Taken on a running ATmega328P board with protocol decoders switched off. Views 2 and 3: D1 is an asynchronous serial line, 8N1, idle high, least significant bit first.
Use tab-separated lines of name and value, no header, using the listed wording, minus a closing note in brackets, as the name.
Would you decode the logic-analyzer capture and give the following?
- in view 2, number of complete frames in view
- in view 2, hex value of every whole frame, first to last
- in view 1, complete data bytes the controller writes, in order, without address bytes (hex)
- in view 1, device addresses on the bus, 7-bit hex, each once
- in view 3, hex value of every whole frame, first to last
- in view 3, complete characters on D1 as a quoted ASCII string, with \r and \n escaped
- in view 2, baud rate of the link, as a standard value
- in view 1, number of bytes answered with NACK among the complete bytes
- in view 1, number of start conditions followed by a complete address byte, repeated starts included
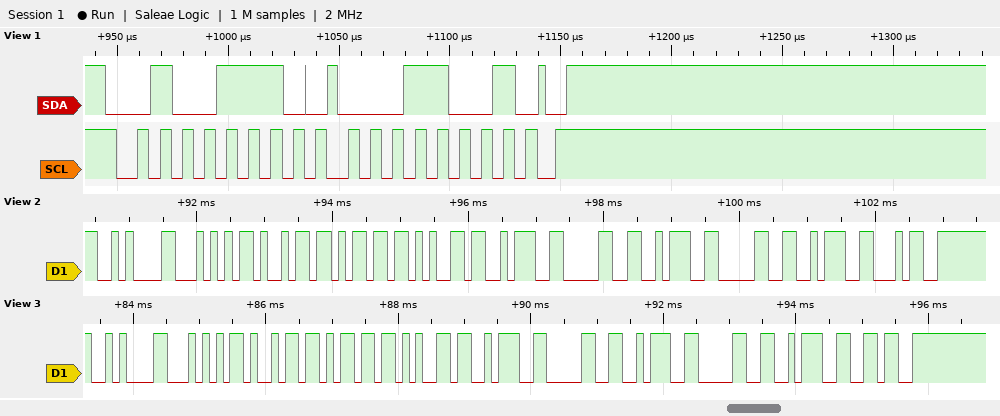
in view 2, number of complete frames in view	11
in view 2, hex value of every whole frame, first to last	0x0A 0x54 0x69 0x6D 0x65 0x3A 0x30 0x3A 0x30 0x3A 0x34
in view 1, complete data bytes the controller writes, in order, without address bytes	19
in view 1, device addresses on the bus, 7-bit hex, each once	0x27
in view 3, hex value of every whole frame, first to last	0x0A 0x54 0x69 0x6D 0x65 0x3A 0x30 0x3A 0x30 0x3A 0x36
in view 3, complete characters on D1 as a quoted ASCII string, with \r and \n escaped	"\nTime:0:0:6"
in view 2, baud rate of the link, as a standard value	9600 baud
in view 1, number of bytes answered with NACK among the complete bytes	0
in view 1, number of start conditions followed by a complete address byte, repeated starts included	1
